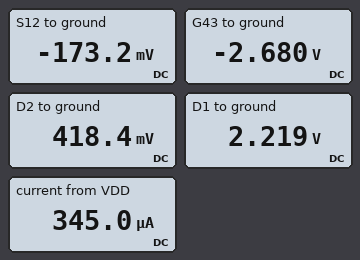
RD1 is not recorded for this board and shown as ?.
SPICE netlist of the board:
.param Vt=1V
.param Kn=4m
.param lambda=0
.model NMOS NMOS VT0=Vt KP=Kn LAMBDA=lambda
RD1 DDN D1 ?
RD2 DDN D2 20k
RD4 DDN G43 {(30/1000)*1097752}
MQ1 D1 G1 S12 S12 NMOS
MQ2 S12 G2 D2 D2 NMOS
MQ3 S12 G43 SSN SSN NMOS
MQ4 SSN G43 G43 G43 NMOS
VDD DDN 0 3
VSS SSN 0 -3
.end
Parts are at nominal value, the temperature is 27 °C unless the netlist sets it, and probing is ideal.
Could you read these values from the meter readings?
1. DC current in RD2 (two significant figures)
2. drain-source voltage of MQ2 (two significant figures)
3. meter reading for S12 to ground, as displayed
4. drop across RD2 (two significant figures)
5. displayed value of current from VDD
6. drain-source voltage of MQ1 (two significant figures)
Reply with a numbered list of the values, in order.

1. 130 µA
2. -590 mV
3. -173.2 mV
4. 2.6 V
5. 345.0 µA
6. 2.4 V
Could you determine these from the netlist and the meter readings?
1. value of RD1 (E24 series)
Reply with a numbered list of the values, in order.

1. 18 kΩ
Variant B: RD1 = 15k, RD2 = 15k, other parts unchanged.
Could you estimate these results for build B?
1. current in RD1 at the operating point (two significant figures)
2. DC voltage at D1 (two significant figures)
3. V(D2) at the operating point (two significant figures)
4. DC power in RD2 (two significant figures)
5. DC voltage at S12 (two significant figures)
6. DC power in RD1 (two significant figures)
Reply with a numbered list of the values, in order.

1. 7.2 µA
2. 2.9 V
3. 520 mV
4. 410 µW
5. -86 mV
6. 790 nW
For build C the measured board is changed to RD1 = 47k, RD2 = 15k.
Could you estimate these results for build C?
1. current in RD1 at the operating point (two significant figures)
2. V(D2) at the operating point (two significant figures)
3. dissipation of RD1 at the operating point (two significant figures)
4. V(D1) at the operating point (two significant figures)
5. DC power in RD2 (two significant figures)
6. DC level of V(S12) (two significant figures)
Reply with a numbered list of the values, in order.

1. 7.2 µA
2. 520 mV
3. 2.5 µW
4. 2.7 V
5. 410 µW
6. -86 mV
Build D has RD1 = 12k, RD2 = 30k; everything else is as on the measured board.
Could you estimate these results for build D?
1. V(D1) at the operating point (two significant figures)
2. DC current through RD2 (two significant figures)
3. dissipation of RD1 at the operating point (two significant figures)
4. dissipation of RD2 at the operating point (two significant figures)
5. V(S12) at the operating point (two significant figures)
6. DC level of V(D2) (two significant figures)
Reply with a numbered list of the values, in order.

1. 2.0 V
2. 90 µA
3. 82 µW
4. 240 µW
5. -230 mV
6. 300 mV
